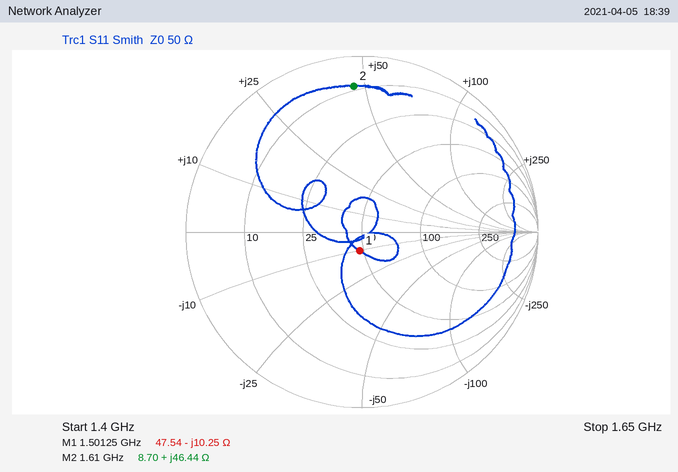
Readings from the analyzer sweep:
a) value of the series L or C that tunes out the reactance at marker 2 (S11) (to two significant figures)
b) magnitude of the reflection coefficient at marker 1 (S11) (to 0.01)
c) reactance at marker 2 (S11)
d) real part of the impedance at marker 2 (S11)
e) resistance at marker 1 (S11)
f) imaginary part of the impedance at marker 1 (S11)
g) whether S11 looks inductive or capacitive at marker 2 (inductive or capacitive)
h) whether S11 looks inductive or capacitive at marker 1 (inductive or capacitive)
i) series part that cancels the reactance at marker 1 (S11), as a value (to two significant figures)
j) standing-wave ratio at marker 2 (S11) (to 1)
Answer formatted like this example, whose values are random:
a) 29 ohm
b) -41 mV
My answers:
a) 2.1 pF
b) 0.11
c) +46.44 Ω
d) 8.70 Ω
e) 47.54 Ω
f) -10.25 Ω
g) inductive
h) capacitive
i) 1.1 nH
j) 11
